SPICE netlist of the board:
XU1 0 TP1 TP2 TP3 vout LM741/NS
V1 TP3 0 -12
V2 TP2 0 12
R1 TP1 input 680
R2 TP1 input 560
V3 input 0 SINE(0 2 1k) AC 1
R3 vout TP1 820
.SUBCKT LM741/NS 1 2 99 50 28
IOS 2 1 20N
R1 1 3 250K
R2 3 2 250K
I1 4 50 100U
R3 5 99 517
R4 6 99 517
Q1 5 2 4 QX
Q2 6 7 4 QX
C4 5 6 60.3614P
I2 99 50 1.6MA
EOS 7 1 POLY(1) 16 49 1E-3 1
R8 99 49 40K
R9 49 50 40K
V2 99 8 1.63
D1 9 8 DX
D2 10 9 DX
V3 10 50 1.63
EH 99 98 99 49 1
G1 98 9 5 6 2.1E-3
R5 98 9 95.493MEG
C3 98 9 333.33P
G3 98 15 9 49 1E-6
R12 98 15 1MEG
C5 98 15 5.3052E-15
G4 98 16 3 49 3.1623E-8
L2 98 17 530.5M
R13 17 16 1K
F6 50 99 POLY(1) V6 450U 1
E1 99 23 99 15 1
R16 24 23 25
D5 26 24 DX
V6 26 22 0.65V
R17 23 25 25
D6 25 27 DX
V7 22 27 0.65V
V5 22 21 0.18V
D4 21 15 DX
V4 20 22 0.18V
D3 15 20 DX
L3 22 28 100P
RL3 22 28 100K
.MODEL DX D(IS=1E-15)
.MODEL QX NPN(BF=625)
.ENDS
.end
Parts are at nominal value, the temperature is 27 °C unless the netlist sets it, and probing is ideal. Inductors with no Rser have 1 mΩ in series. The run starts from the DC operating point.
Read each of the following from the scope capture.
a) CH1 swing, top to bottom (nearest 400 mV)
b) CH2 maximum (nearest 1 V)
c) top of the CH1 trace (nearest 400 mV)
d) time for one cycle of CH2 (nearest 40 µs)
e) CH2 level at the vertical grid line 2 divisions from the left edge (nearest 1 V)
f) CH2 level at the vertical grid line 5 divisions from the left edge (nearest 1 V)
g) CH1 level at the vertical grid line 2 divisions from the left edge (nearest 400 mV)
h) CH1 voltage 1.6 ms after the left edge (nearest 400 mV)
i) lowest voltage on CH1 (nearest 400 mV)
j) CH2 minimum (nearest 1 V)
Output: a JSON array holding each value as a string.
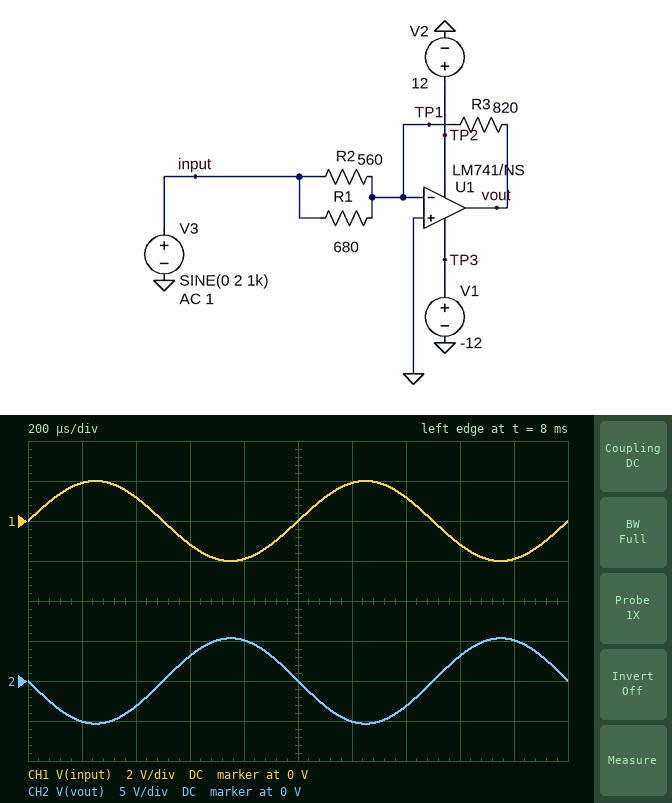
["4.0 V", "5 V", "2.0 V", "1.00 ms", "-3 V", "0 V", "1.2 V", "-1.2 V", "-2.0 V", "-5 V"]
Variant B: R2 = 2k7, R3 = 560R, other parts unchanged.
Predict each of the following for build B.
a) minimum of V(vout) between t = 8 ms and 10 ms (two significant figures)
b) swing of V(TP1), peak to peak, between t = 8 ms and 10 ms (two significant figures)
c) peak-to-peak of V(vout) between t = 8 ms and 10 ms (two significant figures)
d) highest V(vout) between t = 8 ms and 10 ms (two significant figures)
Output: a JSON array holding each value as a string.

["-2.1 V", "5.5 mV", "4.1 V", "2.1 V"]
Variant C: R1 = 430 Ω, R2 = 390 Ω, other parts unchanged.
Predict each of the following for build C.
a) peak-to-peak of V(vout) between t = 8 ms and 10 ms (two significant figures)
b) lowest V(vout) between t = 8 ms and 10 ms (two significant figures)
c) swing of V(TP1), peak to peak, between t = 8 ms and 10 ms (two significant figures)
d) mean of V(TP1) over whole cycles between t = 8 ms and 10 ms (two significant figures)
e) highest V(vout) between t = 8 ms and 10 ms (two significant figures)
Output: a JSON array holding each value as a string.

["16 V", "-8.0 V", "20 mV", "1.0 mV", "8.0 V"]
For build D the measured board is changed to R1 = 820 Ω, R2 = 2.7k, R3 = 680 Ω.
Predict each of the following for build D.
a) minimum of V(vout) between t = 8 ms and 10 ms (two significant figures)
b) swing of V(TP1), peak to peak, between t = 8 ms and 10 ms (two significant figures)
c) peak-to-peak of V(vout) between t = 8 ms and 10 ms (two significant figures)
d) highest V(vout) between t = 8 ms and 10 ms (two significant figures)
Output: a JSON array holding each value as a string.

["-2.2 V", "5.5 mV", "4.3 V", "2.2 V"]
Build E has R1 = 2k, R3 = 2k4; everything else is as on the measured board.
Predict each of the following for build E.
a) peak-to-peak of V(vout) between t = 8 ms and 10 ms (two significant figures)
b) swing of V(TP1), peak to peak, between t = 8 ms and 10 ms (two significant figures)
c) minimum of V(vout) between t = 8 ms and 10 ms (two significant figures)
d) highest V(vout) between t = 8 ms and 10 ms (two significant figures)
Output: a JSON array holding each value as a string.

["22 V", "55 mV", "-11 V", "11 V"]
